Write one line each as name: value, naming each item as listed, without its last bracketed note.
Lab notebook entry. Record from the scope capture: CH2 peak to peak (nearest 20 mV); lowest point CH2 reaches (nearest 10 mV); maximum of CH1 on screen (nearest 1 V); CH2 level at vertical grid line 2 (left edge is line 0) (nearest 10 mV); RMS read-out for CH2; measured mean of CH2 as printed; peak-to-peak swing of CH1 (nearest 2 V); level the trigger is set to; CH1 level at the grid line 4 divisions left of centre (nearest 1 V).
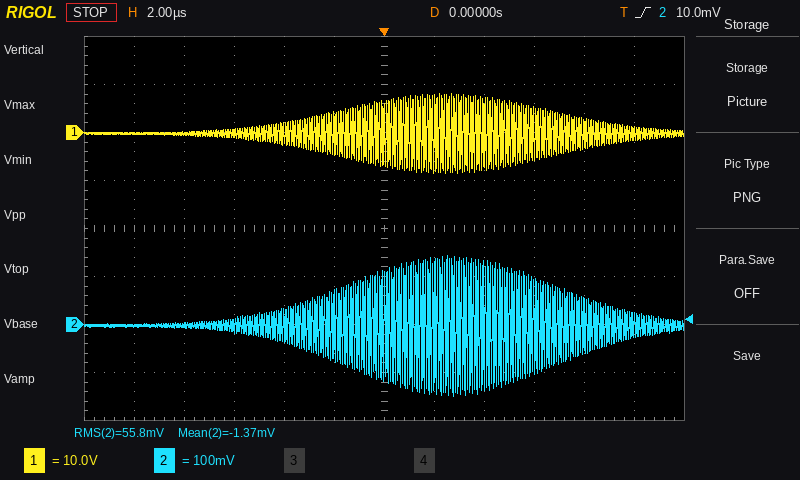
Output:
CH2 peak to peak: 300 mV
lowest point CH2 reaches: -150 mV
maximum of CH1 on screen: 8 V
CH2 level at vertical grid line 2 (left edge is line 0): 0 mV
RMS read-out for CH2: 55.8 mV
measured mean of CH2 as printed: -1.37 mV
peak-to-peak swing of CH1: 16 V
level the trigger is set to: 10.0 mV
CH1 level at the grid line 4 divisions left of centre: 0 V
